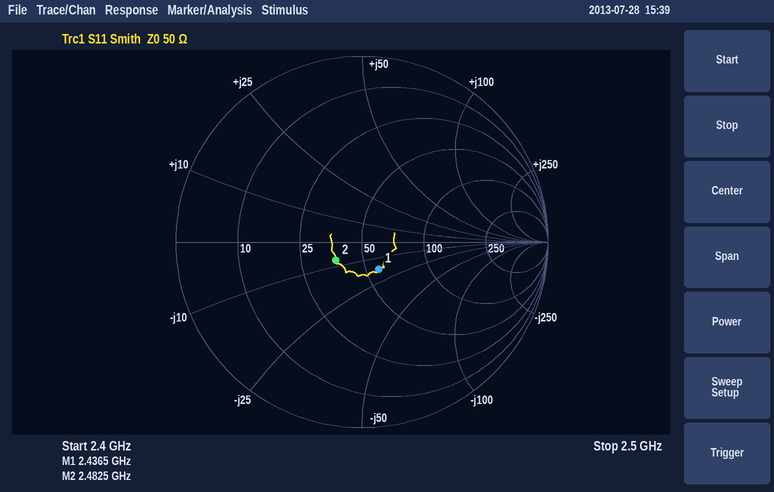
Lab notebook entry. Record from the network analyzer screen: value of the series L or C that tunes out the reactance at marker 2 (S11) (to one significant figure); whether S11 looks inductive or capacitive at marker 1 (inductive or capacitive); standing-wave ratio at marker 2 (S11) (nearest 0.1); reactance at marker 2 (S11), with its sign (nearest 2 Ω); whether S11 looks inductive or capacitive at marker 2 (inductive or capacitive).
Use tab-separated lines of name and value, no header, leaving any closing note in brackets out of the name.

value of the series L or C that tunes out the reactance at marker 2 (S11)	500 pH
whether S11 looks inductive or capacitive at marker 1	capacitive
standing-wave ratio at marker 2 (S11)	1.4
reactance at marker 2 (S11), with its sign	-8 Ω
whether S11 looks inductive or capacitive at marker 2	capacitive
